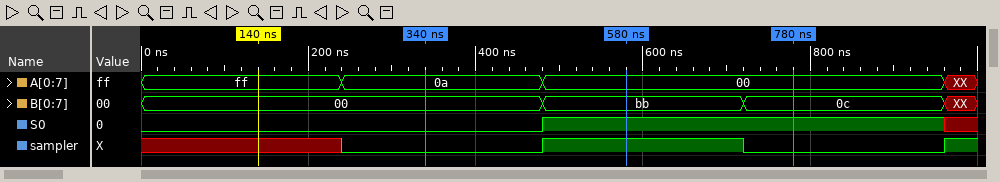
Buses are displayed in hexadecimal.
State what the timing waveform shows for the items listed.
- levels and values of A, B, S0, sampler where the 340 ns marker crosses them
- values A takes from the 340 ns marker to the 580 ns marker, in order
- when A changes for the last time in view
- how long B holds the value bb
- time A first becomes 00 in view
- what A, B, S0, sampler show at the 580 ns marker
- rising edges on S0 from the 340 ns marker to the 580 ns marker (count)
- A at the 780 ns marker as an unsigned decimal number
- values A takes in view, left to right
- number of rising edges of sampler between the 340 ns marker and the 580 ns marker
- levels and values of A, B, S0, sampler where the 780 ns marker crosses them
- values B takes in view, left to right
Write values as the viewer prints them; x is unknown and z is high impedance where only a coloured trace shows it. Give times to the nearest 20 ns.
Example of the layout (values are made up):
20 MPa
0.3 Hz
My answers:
A=0a, B=00, S0=0, sampler=0
0a, 00
960 ns
240 ns
480 ns
A=00, B=bb, S0=1, sampler=1
1
0
ff, 0a, 00, XX
1
A=00, B=0c, S0=1, sampler=0
00, bb, 0c, XX
